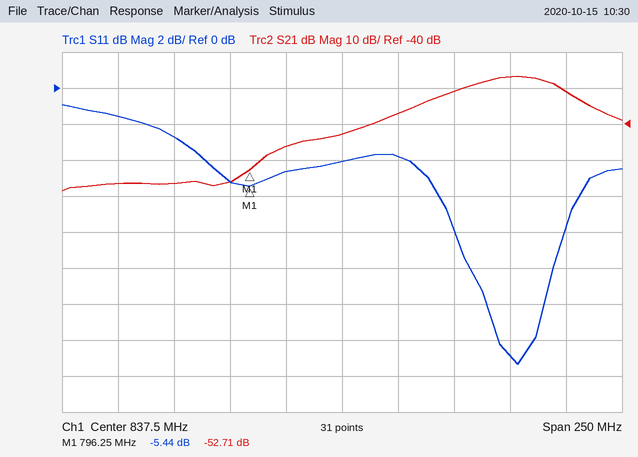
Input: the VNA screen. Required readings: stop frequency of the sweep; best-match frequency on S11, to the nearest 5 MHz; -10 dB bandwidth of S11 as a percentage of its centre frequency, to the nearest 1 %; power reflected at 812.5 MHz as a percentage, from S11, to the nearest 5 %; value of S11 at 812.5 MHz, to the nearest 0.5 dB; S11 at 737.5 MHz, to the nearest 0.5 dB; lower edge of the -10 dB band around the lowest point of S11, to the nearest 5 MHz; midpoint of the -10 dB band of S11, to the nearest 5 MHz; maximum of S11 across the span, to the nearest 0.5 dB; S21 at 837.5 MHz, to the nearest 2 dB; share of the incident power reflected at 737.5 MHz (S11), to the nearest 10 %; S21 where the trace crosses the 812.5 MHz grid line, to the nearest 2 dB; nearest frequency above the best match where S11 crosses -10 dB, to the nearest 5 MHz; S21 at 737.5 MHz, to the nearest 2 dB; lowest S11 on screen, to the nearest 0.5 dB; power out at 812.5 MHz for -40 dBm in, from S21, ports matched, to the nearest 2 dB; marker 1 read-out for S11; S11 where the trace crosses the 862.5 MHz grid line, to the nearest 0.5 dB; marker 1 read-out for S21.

962.5 MHz
915 MHz
4 %
35 %
-4.5 dB
-1.5 dB
895 MHz
915 MHz
-1.0 dB
-42 dB
70 %
-46 dB
930 MHz
-56 dB
-15.5 dB
-86 dBm
-5.44 dB
-4.0 dB
-52.71 dB
